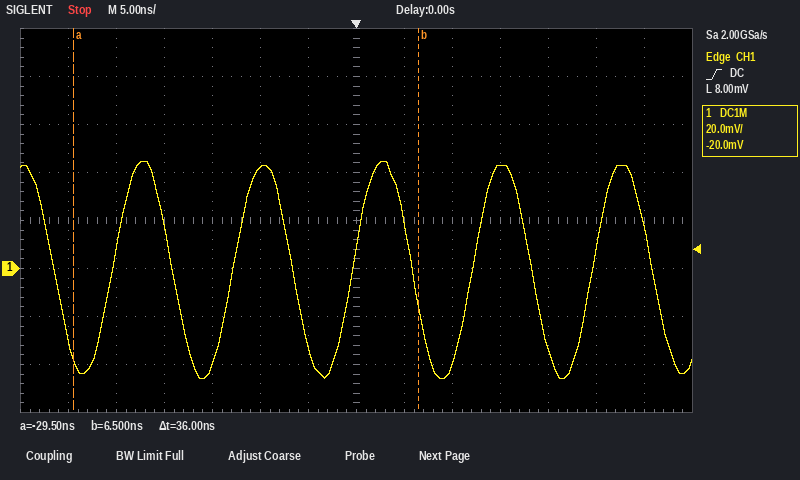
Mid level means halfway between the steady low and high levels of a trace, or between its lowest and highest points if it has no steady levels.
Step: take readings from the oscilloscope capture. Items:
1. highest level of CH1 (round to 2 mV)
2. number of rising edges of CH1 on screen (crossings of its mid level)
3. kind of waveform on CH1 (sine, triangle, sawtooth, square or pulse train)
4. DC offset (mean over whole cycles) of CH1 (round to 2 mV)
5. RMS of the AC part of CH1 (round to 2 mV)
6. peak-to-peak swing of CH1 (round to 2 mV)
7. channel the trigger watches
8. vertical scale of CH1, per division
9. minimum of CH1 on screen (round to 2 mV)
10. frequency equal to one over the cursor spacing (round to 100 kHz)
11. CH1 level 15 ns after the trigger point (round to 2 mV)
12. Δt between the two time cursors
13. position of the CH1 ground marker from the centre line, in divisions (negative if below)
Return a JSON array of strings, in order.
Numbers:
["44 mV", "5", "sine", "0 mV", "32 mV", "90 mV", "CH1", "20 mV", "-46 mV", "27.8 MHz", "42 mV", "36 ns", "-1.0 div"]
